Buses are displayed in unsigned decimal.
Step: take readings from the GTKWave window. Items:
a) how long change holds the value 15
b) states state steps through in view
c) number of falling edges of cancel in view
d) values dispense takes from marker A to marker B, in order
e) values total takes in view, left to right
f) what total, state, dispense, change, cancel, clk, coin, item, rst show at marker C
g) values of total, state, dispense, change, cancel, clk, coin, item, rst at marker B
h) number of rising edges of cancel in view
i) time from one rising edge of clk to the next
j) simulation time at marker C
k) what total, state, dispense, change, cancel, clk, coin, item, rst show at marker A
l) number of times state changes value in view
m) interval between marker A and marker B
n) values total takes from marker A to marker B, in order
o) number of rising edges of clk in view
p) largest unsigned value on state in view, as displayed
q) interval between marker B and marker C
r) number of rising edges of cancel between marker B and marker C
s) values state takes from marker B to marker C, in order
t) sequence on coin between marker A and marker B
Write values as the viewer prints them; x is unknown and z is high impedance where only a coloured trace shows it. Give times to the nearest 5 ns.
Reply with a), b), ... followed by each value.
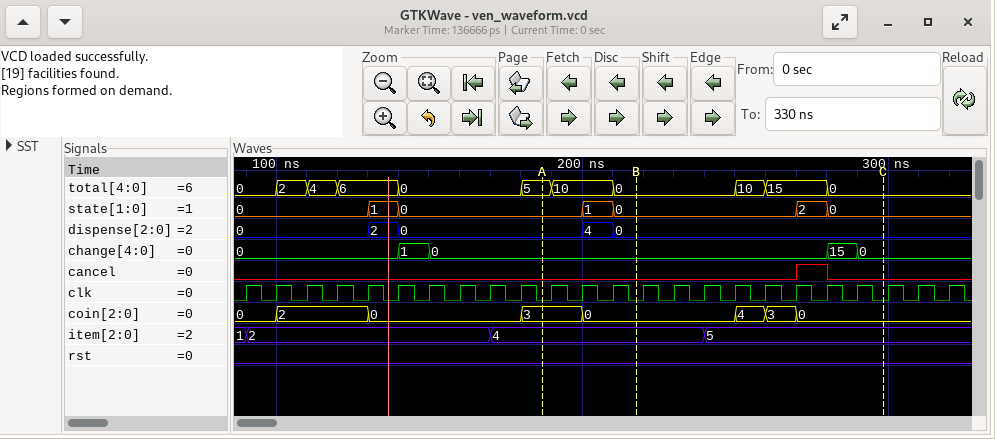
a) 10 ns
b) 0, 1, 0, 1, 0, 2, 0
c) 1
d) 0, 4, 0
e) 0, 2, 4, 6, 0, 5, 10, 0, 10, 15, 0
f) total=0, state=0, dispense=0, change=0, cancel=0, clk=0, coin=0, item=5, rst=0
g) total=0, state=0, dispense=0, change=0, cancel=0, clk=0, coin=0, item=4, rst=0
h) 1
i) 10 ns
j) 300 ns
k) total=5, state=0, dispense=0, change=0, cancel=0, clk=0, coin=3, item=4, rst=0
l) 6
m) 30 ns
n) 5, 10, 0
o) 24
p) 2
q) 80 ns
r) 1
s) 0, 2, 0
t) 3, 0
